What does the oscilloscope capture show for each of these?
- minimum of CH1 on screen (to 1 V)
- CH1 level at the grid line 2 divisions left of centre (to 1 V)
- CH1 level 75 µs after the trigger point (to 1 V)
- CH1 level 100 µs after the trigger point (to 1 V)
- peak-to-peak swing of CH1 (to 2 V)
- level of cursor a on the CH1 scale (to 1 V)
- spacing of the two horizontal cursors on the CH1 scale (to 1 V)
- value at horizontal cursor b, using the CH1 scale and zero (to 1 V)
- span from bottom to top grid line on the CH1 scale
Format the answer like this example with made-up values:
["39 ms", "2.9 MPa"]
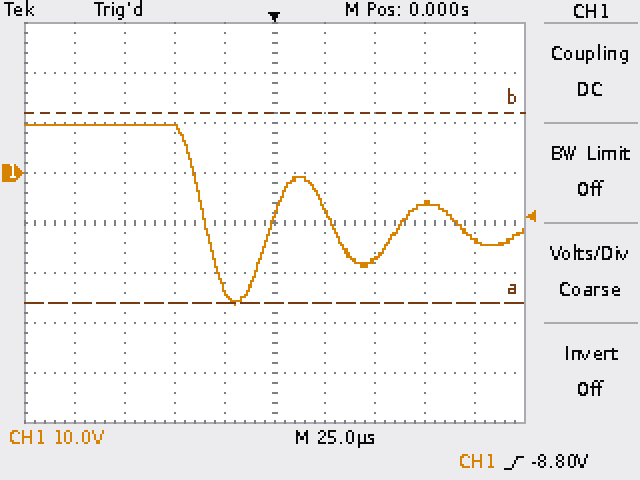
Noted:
["-26 V", "9 V", "-6 V", "-13 V", "36 V", "-26 V", "38 V", "12 V", "80 V"]
